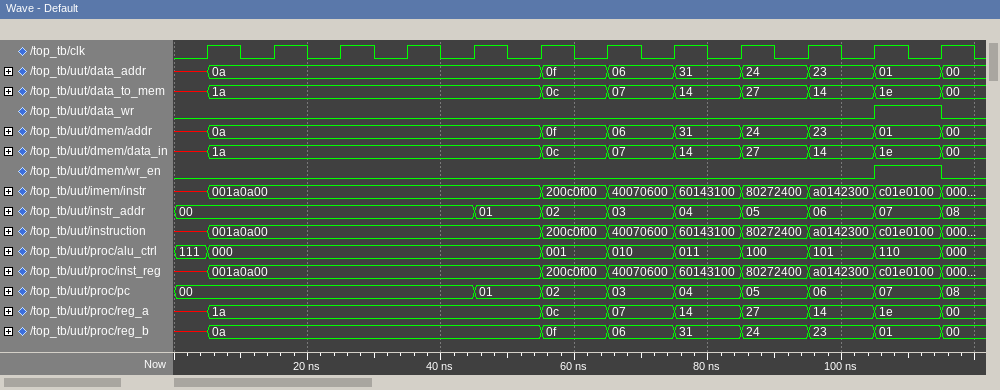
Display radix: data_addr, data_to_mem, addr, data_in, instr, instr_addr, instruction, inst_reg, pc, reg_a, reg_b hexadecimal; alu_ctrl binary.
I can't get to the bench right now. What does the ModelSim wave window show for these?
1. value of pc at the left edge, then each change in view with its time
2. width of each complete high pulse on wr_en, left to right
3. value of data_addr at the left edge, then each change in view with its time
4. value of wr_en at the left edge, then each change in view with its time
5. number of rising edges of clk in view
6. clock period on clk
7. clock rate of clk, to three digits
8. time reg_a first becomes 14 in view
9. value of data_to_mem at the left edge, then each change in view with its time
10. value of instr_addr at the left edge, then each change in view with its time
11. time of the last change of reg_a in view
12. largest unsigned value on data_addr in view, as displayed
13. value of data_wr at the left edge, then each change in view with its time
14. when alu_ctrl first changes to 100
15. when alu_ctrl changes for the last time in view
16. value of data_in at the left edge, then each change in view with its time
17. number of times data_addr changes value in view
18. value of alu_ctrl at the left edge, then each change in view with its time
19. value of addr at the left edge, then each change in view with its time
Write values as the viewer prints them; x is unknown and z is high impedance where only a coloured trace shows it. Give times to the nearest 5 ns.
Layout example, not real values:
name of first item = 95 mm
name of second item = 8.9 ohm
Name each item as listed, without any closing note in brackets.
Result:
value of pc at the left edge, then each change in view with its time = 00, 01 at 45 ns, 02 at 55 ns, 03 at 65 ns, 04 at 75 ns, 05 at 85 ns, 06 at 95 ns, 07 at 105 ns, 08 at 115 ns
width of each complete high pulse on wr_en, left to right = 10 ns
value of data_addr at the left edge, then each change in view with its time = x, 0a at 5 ns, 0f at 55 ns, 06 at 65 ns, 31 at 75 ns, 24 at 85 ns, 23 at 95 ns, 01 at 105 ns, 00 at 115 ns
value of wr_en at the left edge, then each change in view with its time = 0, 1 at 105 ns, 0 at 115 ns
number of rising edges of clk in view = 12
clock period on clk = 10 ns
clock rate of clk, to three digits = 100 MHz
time reg_a first becomes 14 in view = 75 ns
value of data_to_mem at the left edge, then each change in view with its time = x, 1a at 5 ns, 0c at 55 ns, 07 at 65 ns, 14 at 75 ns, 27 at 85 ns, 14 at 95 ns, 1e at 105 ns, 00 at 115 ns
value of instr_addr at the left edge, then each change in view with its time = 00, 01 at 45 ns, 02 at 55 ns, 03 at 65 ns, 04 at 75 ns, 05 at 85 ns, 06 at 95 ns, 07 at 105 ns, 08 at 115 ns
time of the last change of reg_a in view = 115 ns
largest unsigned value on data_addr in view, as displayed = 31
value of data_wr at the left edge, then each change in view with its time = 0, 1 at 105 ns, 0 at 115 ns
when alu_ctrl first changes to 100 = 85 ns
when alu_ctrl changes for the last time in view = 115 ns
value of data_in at the left edge, then each change in view with its time = x, 1a at 5 ns, 0c at 55 ns, 07 at 65 ns, 14 at 75 ns, 27 at 85 ns, 14 at 95 ns, 1e at 105 ns, 00 at 115 ns
number of times data_addr changes value in view = 8
value of alu_ctrl at the left edge, then each change in view with its time = 111, 000 at 5 ns, 001 at 55 ns, 010 at 65 ns, 011 at 75 ns, 100 at 85 ns, 101 at 95 ns, 110 at 105 ns, 000 at 115 ns
value of addr at the left edge, then each change in view with its time = x, 0a at 5 ns, 0f at 55 ns, 06 at 65 ns, 31 at 75 ns, 24 at 85 ns, 23 at 95 ns, 01 at 105 ns, 00 at 115 ns
